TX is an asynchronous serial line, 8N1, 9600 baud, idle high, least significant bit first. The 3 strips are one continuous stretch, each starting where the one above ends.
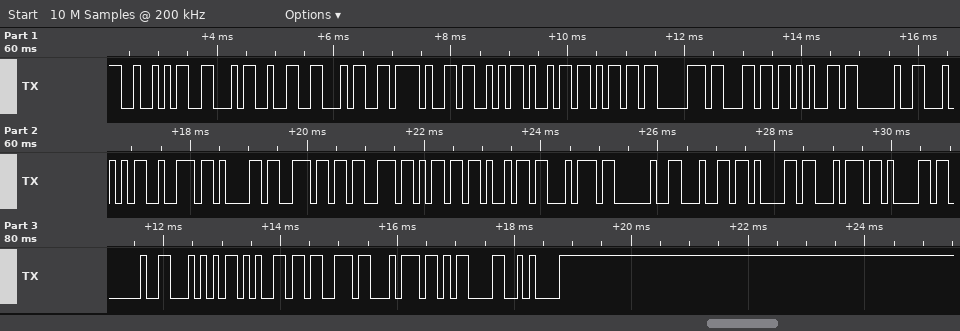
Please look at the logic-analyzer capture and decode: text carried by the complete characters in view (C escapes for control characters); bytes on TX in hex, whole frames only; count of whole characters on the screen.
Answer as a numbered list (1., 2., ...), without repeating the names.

1. "RF24/Simple Transmit data Test\r\n"
2. 0x52 0x46 0x32 0x34 0x2F 0x53 0x69 0x6D 0x70 0x6C 0x65 0x20 0x54 0x72 0x61 0x6E 0x73 0x6D 0x69 0x74 0x20 0x64 0x61 0x74 0x61 0x20 0x54 0x65 0x73 0x74 0x0D 0x0A
3. 32
